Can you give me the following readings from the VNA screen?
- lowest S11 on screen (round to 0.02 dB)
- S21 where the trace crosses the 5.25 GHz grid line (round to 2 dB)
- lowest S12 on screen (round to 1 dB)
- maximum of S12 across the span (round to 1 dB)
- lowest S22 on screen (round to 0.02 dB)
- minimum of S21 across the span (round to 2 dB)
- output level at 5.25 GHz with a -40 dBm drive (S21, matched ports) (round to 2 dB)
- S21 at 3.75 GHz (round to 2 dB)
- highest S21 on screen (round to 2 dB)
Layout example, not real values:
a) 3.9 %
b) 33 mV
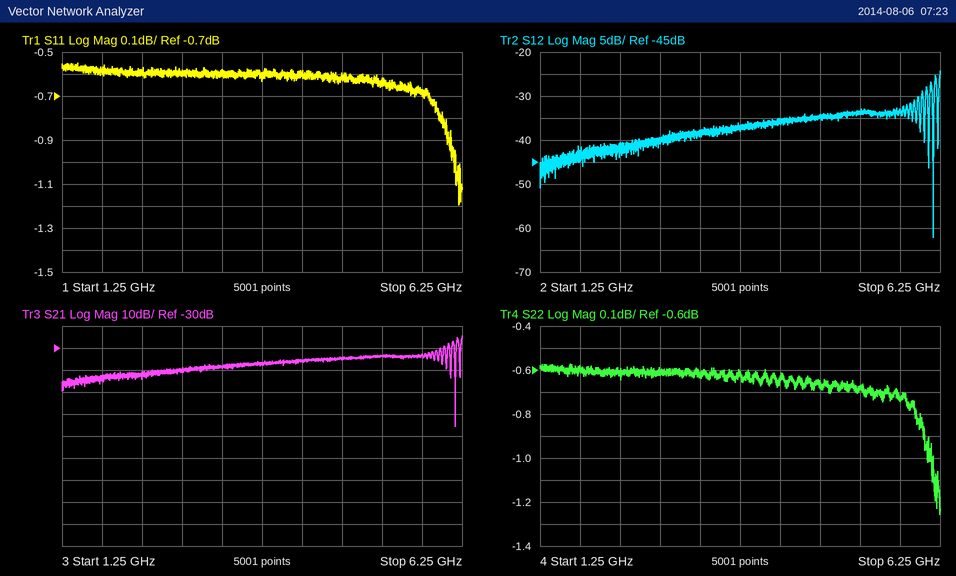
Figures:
a) -1.20 dB
b) -34 dB
c) -62 dB
d) -24 dB
e) -1.26 dB
f) -66 dB
g) -74 dBm
h) -38 dB
i) -24 dB
